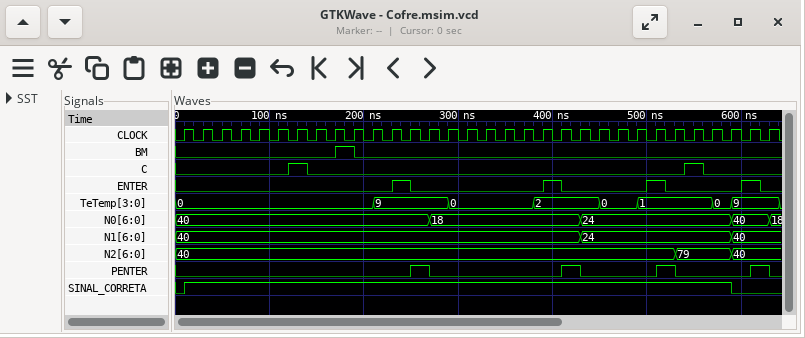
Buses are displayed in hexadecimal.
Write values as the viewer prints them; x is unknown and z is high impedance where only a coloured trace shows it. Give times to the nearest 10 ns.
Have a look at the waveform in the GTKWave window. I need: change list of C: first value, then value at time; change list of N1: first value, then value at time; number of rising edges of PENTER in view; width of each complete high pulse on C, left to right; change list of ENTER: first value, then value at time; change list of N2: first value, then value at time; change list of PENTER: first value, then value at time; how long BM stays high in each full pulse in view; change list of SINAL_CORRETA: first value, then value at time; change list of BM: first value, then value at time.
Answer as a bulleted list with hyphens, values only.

- 0, 1 at 120 ns, 0 at 140 ns, 1 at 540 ns, 0 at 560 ns
- 40, 24 at 430 ns, 40 at 590 ns
- 4
- 20 ns, 20 ns
- 0, 1 at 230 ns, 0 at 250 ns, 1 at 390 ns, 0 at 410 ns, 1 at 500 ns, 0 at 520 ns, 1 at 600 ns, 0 at 620 ns
- 40, 79 at 530 ns, 40 at 590 ns
- 0, 1 at 250 ns, 0 at 270 ns, 1 at 410 ns, 0 at 430 ns, 1 at 510 ns, 0 at 530 ns, 1 at 610 ns, 0 at 630 ns
- 20 ns
- 0, 1 at 10 ns, 0 at 590 ns
- 0, 1 at 170 ns, 0 at 190 ns
